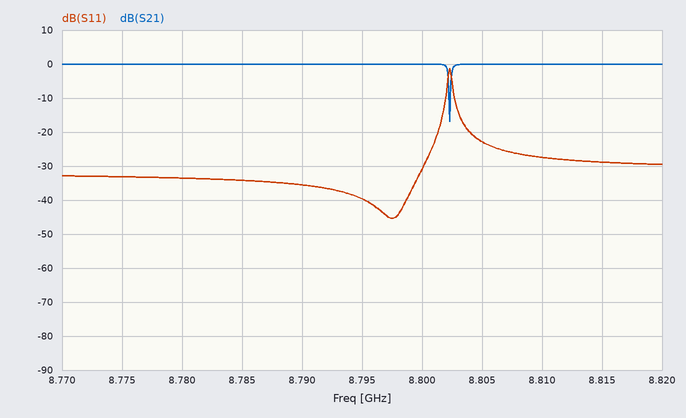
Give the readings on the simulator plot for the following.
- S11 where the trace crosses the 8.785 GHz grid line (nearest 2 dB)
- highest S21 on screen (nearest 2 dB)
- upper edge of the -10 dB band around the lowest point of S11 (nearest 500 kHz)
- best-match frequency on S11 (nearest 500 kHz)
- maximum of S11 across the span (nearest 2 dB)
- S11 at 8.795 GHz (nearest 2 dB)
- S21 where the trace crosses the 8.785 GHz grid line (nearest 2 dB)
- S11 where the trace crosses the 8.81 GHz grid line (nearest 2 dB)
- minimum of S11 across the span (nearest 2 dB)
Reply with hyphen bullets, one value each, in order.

- -34 dB
- 0 dB
- 8.8020 GHz
- 8.7975 GHz
- -2 dB
- -40 dB
- 0 dB
- -28 dB
- -46 dB
